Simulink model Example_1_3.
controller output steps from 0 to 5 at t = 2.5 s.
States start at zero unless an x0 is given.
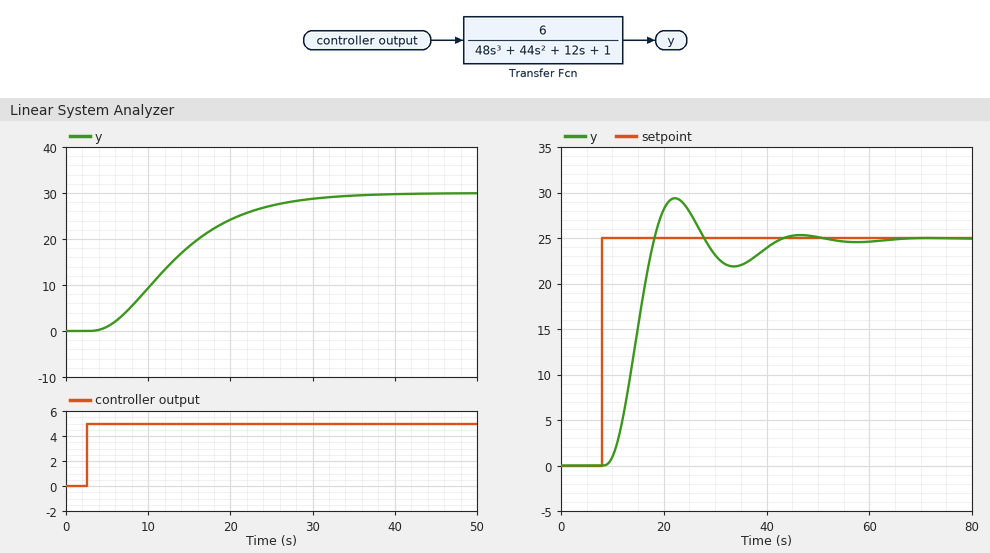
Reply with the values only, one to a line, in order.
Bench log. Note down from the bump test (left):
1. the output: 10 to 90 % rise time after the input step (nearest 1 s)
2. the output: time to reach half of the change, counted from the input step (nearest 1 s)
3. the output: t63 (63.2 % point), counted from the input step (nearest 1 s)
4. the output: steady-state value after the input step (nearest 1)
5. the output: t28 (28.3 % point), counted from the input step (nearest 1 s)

18 s
10 s
13 s
30
7 s
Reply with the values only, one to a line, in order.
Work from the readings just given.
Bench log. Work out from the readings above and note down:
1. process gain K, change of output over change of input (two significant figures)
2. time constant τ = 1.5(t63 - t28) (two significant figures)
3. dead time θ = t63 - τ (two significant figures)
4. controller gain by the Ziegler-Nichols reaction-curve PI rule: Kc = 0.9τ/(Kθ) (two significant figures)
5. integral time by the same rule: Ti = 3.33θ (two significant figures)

6.0
9.0 s
4.0 s
0.34
13 s
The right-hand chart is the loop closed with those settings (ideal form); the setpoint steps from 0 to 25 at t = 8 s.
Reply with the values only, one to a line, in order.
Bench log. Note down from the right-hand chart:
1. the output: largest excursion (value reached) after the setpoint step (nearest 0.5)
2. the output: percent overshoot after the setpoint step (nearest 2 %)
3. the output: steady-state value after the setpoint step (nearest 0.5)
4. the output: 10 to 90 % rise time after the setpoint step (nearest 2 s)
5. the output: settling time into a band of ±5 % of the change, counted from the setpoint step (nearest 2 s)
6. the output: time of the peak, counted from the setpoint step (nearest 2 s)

29.5
18 %
25.0
6 s
32 s
14 s
